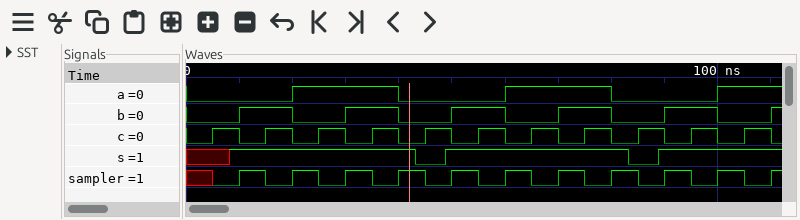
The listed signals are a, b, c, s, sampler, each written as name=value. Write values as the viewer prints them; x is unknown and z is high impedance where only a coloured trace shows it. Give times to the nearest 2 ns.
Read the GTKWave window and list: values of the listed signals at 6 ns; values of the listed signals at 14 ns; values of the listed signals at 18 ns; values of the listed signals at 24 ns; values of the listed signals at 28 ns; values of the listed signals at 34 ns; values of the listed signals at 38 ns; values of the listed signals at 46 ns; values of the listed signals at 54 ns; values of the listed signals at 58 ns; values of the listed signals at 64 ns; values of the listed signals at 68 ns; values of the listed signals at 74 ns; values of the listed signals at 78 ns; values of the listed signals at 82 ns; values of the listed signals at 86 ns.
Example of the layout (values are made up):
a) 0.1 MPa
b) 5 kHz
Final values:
a) a=0, b=0, c=1, s=x, sampler=0
b) a=0, b=1, c=0, s=1, sampler=1
c) a=0, b=1, c=1, s=1, sampler=0
d) a=1, b=0, c=0, s=1, sampler=1
e) a=1, b=0, c=1, s=1, sampler=0
f) a=1, b=1, c=0, s=1, sampler=1
g) a=1, b=1, c=1, s=1, sampler=0
h) a=0, b=0, c=1, s=0, sampler=0
i) a=0, b=1, c=0, s=1, sampler=1
j) a=0, b=1, c=1, s=1, sampler=0
k) a=1, b=0, c=0, s=1, sampler=1
l) a=1, b=0, c=1, s=1, sampler=0
m) a=1, b=1, c=0, s=1, sampler=1
n) a=1, b=1, c=1, s=1, sampler=0
o) a=0, b=0, c=0, s=1, sampler=1
p) a=0, b=0, c=1, s=0, sampler=0
